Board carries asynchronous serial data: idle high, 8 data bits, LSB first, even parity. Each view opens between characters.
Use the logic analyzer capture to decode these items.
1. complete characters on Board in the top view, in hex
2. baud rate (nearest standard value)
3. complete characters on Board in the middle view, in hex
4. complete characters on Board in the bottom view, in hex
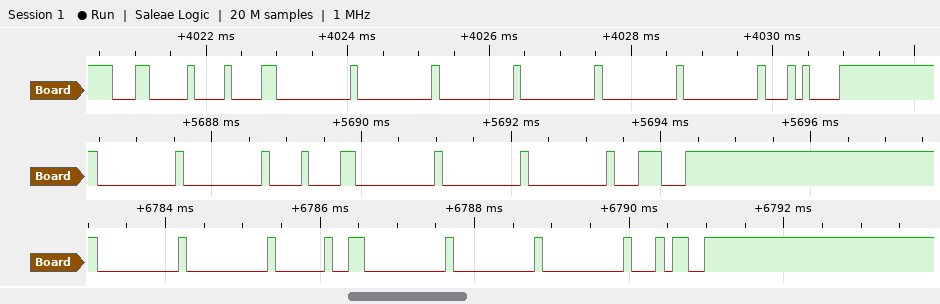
0C, 08, 00, 00, 00, 00, 00, 00, 14
9600 baud
00, 00, 08, 00, 00, 00, 1C
00, 00, 20, 00, 00, 00, 34
